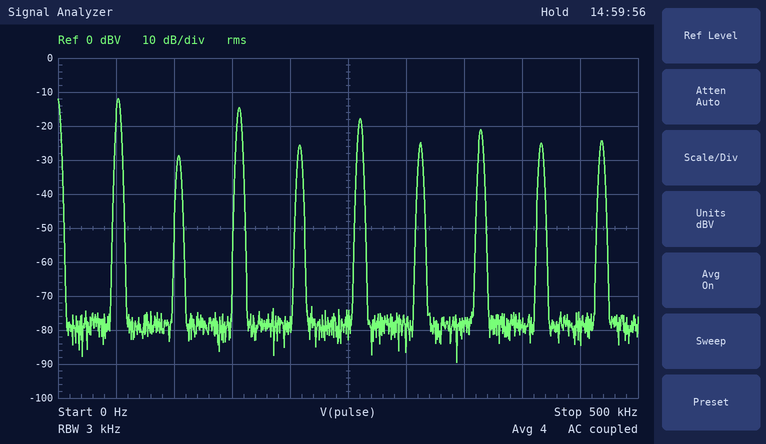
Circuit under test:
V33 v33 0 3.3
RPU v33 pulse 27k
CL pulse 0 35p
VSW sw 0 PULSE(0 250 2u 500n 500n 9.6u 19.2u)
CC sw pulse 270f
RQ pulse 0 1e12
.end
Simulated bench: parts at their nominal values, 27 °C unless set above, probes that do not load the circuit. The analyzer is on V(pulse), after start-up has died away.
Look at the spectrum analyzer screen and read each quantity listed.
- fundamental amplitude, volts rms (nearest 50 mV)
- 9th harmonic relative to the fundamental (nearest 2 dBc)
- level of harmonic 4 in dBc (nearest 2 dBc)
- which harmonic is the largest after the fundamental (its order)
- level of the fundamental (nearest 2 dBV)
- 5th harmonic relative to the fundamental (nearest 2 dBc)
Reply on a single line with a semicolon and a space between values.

250 mV; -12 dBc; -14 dBc; 3; -12 dBV; -6 dBc
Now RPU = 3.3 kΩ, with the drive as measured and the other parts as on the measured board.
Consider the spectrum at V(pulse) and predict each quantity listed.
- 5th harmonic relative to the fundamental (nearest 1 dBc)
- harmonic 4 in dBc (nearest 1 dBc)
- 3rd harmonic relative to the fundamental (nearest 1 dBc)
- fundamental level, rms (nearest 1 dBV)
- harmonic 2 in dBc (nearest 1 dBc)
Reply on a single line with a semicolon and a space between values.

-1 dBc; -10 dBc; 0 dBc; -30 dBV; -16 dBc
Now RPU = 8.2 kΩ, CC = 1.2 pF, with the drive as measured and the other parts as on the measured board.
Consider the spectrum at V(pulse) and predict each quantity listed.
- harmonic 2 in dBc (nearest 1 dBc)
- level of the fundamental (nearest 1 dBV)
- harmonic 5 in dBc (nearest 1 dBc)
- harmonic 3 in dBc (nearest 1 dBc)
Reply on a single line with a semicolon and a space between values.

-16 dBc; -9 dBV; -2 dBc; -1 dBc
